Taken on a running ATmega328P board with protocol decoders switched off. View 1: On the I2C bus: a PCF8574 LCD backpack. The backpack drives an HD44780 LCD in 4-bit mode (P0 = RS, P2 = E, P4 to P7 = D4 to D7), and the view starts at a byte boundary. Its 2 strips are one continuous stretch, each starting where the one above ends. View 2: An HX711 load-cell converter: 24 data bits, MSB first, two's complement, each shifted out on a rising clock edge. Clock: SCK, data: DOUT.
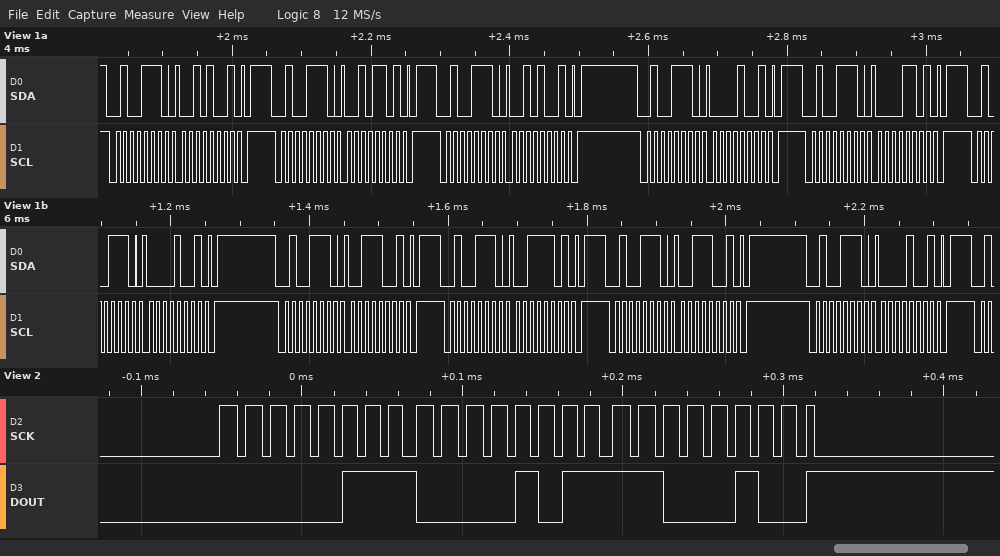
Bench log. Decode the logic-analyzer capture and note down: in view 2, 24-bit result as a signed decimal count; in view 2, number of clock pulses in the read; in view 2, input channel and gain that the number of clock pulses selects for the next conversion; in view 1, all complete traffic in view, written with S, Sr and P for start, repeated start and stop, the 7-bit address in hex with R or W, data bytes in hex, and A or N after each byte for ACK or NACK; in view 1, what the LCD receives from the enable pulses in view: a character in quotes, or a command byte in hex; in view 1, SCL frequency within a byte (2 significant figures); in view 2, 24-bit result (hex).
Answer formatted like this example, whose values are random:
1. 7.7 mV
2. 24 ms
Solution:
1. 461764
2. 25
3. channel A, gain 128
4. S 27W A 29 A P S 27W A 2D A P S 27W A 29 A P S 27W A 09 A P S 27W A 0D A P S 27W A 09 A P S 27W A 39 A P S 27W A 3D A P S 27W A 39 A P S 27W A 09 A P
5. ' '
6. 100 kHz
7. 0x070BC4
